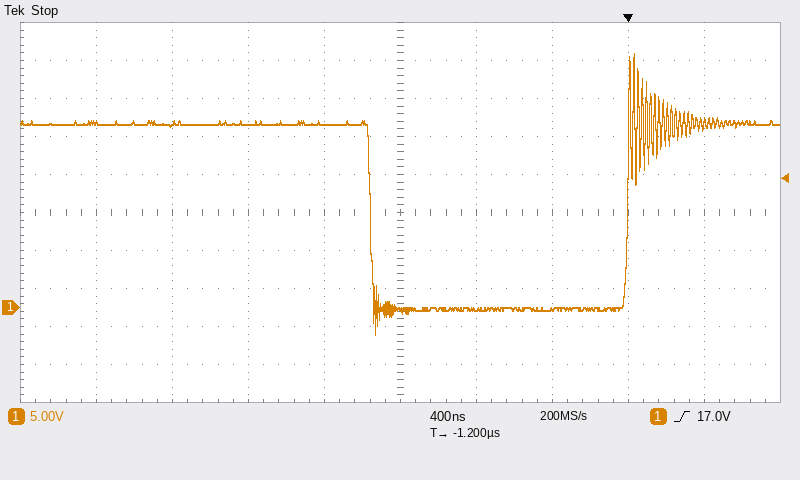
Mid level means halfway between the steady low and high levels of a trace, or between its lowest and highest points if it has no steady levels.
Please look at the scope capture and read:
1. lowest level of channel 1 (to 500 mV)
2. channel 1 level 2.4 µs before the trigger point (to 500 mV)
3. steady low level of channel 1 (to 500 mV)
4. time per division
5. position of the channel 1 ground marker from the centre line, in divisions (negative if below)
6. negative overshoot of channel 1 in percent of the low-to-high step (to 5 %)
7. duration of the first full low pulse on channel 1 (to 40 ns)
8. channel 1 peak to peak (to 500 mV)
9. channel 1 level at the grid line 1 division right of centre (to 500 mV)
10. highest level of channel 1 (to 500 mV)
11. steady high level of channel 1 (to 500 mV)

-3.5 V
24.0 V
0.0 V
400 ns
-2.5 div
15 %
1.36 µs
37.0 V
0.0 V
33.5 V
24.0 V
